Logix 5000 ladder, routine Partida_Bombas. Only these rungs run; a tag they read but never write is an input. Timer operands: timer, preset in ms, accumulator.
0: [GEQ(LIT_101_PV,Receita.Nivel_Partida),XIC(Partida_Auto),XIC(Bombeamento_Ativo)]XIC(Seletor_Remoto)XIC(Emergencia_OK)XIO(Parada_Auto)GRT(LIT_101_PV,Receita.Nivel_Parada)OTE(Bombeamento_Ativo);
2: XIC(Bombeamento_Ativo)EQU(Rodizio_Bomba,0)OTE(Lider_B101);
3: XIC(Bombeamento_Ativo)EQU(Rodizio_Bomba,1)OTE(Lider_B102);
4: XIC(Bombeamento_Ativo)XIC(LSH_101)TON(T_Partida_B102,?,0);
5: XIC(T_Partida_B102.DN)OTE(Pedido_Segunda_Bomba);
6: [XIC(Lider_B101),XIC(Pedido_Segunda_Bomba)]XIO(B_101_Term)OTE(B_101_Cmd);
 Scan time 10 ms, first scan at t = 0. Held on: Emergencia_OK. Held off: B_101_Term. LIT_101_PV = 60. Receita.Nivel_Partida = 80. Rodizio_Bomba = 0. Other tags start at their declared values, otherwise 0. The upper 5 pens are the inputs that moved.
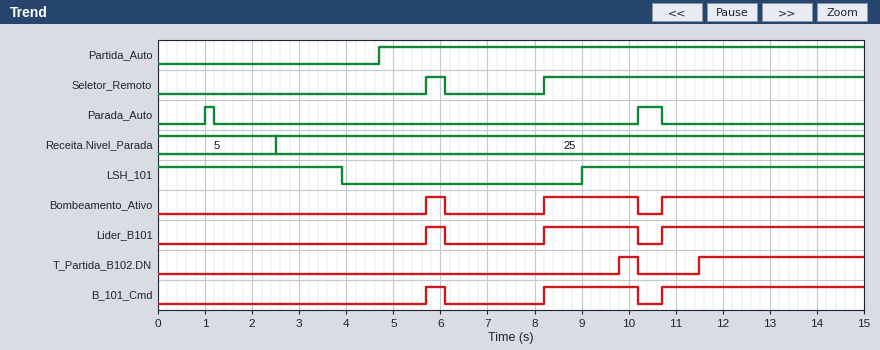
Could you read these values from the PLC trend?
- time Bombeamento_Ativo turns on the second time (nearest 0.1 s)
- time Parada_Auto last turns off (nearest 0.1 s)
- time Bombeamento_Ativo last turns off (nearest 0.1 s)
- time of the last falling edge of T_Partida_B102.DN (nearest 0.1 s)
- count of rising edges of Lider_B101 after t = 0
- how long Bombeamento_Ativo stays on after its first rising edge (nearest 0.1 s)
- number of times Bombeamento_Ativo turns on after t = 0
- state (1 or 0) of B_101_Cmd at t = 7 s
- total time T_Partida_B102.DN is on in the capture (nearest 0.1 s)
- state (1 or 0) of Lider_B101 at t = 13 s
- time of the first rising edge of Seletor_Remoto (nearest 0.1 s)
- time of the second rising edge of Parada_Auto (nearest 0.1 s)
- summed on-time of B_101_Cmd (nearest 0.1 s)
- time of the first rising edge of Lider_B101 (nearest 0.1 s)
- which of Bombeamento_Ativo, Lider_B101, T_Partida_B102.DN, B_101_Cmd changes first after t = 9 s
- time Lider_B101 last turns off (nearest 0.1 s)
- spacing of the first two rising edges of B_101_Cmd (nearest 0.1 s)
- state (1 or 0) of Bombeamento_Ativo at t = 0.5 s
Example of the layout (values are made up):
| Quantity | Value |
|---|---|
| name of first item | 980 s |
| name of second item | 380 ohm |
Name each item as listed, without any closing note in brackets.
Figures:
| Quantity | Value |
|---|---|
| time Bombeamento_Ativo turns on the second time | 8.2 s |
| time Parada_Auto last turns off | 10.7 s |
| time Bombeamento_Ativo last turns off | 10.2 s |
| time of the last falling edge of T_Partida_B102.DN | 10.2 s |
| count of rising edges of Lider_B101 after t = 0 | 3 |
| how long Bombeamento_Ativo stays on after its first rising edge | 0.4 s |
| number of times Bombeamento_Ativo turns on after t = 0 | 3 |
| state (1 or 0) of B_101_Cmd at t = 7 s | 0 |
| total time T_Partida_B102.DN is on in the capture | 3.9 s |
| state (1 or 0) of Lider_B101 at t = 13 s | 1 |
| time of the first rising edge of Seletor_Remoto | 5.7 s |
| time of the second rising edge of Parada_Auto | 10.2 s |
| summed on-time of B_101_Cmd | 6.7 s |
| time of the first rising edge of Lider_B101 | 5.7 s |
| which of Bombeamento_Ativo, Lider_B101, T_Partida_B102.DN, B_101_Cmd changes first after t = 9 s | T_Partida_B102.DN |
| time Lider_B101 last turns off | 10.2 s |
| spacing of the first two rising edges of B_101_Cmd | 2.5 s |
| state (1 or 0) of Bombeamento_Ativo at t = 0.5 s | 0 |
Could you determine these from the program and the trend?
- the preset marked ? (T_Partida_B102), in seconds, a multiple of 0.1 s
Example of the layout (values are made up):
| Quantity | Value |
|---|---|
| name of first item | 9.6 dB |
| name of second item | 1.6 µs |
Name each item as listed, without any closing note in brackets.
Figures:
| Quantity | Value |
|---|---|
| the preset marked ? (T_Partida_B102), in seconds, a multiple of 0.1 s | 0.8 s |
